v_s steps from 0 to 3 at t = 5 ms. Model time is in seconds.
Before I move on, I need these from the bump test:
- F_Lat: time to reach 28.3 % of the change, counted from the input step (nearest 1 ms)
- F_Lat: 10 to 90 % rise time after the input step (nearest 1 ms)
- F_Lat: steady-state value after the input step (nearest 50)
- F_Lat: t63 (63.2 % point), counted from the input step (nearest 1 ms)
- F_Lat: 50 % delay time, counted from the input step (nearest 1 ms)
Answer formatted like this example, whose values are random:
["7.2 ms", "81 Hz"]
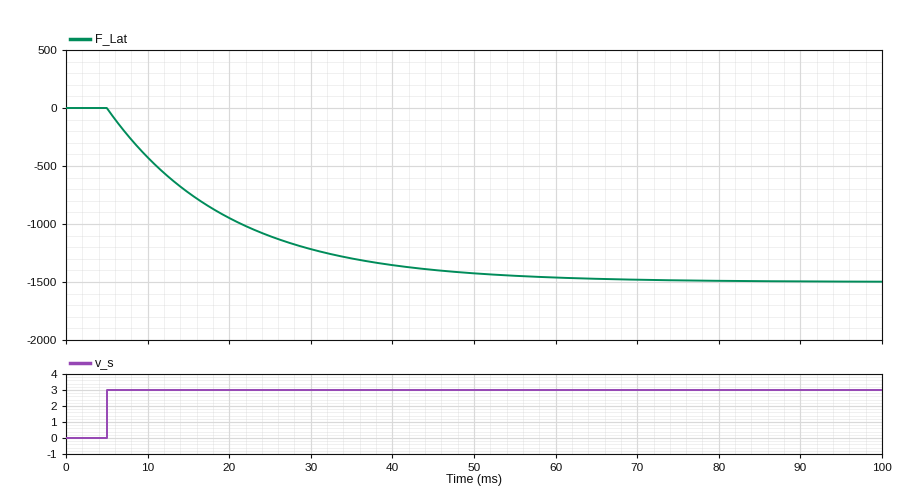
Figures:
["5 ms", "33 ms", "-1500", "15 ms", "10 ms"]
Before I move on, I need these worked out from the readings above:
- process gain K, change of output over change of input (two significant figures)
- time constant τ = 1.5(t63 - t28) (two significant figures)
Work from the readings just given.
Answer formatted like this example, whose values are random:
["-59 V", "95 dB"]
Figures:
["-500", "15 ms"]
